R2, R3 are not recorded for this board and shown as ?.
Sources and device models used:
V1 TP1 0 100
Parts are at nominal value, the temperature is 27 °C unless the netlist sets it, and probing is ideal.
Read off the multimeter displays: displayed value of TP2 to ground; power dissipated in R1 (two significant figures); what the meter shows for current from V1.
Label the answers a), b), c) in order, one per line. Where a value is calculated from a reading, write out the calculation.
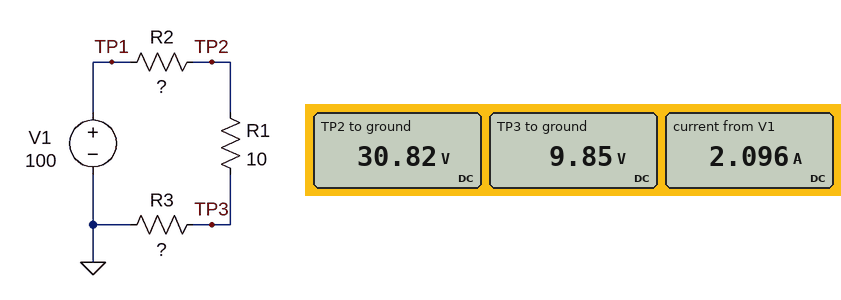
a) 30.82 V
b) (30.82 V - 9.85 V)^2 / 10 Ω = 44 W
c) 2.096 A
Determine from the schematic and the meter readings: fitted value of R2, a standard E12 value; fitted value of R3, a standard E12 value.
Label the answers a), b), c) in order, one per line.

a) 33 Ω
b) 4.7 Ω
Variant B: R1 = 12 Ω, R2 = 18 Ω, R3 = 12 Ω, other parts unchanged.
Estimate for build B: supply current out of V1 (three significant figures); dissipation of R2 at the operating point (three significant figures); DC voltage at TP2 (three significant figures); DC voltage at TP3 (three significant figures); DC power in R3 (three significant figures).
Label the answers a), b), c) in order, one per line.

a) 2.38 A
b) 102 W
c) 57.1 V
d) 28.6 V
e) 68.0 W
